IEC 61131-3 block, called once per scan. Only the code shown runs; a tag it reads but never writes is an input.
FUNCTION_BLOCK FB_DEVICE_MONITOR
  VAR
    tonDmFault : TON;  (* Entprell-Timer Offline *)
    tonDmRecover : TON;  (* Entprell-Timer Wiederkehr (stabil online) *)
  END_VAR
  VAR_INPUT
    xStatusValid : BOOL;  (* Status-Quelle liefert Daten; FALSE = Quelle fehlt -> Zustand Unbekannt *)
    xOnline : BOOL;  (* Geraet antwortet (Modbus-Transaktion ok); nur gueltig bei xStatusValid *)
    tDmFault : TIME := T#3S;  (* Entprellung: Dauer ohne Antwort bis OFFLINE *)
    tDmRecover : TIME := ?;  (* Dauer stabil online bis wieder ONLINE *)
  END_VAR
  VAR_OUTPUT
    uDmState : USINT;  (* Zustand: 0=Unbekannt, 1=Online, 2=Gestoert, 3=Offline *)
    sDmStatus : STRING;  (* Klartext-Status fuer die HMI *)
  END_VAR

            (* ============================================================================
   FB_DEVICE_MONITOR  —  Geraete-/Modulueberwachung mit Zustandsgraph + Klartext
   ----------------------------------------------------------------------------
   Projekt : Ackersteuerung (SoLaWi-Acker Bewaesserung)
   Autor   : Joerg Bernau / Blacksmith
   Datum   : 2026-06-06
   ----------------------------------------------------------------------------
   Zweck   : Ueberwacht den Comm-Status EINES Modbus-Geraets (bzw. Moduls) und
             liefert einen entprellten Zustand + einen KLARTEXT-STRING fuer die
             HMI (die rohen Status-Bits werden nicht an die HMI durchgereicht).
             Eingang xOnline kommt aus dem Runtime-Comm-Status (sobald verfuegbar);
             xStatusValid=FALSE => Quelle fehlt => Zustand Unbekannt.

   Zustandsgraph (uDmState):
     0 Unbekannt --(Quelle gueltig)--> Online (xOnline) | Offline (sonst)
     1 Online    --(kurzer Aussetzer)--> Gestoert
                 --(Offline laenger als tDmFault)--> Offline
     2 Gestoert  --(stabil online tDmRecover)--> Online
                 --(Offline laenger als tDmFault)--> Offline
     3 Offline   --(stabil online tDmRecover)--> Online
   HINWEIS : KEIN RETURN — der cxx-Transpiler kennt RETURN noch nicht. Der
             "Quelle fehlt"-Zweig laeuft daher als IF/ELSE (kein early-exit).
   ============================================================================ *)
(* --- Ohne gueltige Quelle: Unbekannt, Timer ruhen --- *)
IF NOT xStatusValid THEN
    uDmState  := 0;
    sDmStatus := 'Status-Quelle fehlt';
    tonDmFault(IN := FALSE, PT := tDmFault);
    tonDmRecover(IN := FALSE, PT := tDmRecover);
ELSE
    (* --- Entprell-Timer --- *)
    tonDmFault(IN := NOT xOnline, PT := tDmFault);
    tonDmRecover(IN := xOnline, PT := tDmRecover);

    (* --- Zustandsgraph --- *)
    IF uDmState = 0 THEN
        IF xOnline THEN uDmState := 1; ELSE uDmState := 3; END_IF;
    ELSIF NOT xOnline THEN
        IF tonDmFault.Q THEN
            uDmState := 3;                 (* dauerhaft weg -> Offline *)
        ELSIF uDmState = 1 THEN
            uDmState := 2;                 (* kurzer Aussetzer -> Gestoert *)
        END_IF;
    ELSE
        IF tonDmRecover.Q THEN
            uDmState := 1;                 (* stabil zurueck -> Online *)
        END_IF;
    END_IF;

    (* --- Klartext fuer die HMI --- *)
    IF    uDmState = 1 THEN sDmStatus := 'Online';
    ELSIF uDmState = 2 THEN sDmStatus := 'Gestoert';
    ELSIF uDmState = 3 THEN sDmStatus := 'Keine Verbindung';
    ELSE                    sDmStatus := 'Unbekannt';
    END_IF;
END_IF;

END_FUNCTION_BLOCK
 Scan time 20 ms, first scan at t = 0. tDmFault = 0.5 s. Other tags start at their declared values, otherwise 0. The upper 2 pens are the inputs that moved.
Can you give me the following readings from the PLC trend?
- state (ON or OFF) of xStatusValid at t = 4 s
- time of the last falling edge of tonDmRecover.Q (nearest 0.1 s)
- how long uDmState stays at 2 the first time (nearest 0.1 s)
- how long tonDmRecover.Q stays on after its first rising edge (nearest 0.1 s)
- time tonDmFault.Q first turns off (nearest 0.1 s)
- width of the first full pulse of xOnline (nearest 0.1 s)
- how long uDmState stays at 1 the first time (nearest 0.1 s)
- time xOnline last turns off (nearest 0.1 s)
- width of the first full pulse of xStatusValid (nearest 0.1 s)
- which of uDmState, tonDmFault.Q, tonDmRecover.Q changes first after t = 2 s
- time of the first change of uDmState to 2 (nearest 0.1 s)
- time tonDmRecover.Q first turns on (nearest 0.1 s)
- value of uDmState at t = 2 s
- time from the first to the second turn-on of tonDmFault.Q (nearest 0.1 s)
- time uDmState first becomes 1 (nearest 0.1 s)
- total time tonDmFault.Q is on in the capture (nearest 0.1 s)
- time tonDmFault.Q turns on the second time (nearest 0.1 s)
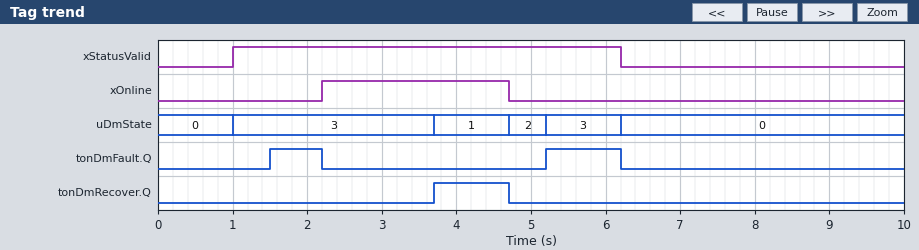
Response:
ON
4.7 s
0.5 s
1.0 s
2.2 s
2.5 s
1.0 s
4.7 s
5.2 s
tonDmFault.Q
4.7 s
3.7 s
3
3.7 s
3.7 s
1.7 s
5.2 s
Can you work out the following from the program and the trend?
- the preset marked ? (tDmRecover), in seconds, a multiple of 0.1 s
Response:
1.5 s
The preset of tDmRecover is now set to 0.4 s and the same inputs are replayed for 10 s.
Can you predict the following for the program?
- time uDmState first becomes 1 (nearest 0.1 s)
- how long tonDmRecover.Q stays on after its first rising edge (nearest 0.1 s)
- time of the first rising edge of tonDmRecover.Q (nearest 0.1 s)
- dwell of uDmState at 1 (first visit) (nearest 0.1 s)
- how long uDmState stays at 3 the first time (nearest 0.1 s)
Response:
2.6 s
2.1 s
2.6 s
2.1 s
1.6 s
